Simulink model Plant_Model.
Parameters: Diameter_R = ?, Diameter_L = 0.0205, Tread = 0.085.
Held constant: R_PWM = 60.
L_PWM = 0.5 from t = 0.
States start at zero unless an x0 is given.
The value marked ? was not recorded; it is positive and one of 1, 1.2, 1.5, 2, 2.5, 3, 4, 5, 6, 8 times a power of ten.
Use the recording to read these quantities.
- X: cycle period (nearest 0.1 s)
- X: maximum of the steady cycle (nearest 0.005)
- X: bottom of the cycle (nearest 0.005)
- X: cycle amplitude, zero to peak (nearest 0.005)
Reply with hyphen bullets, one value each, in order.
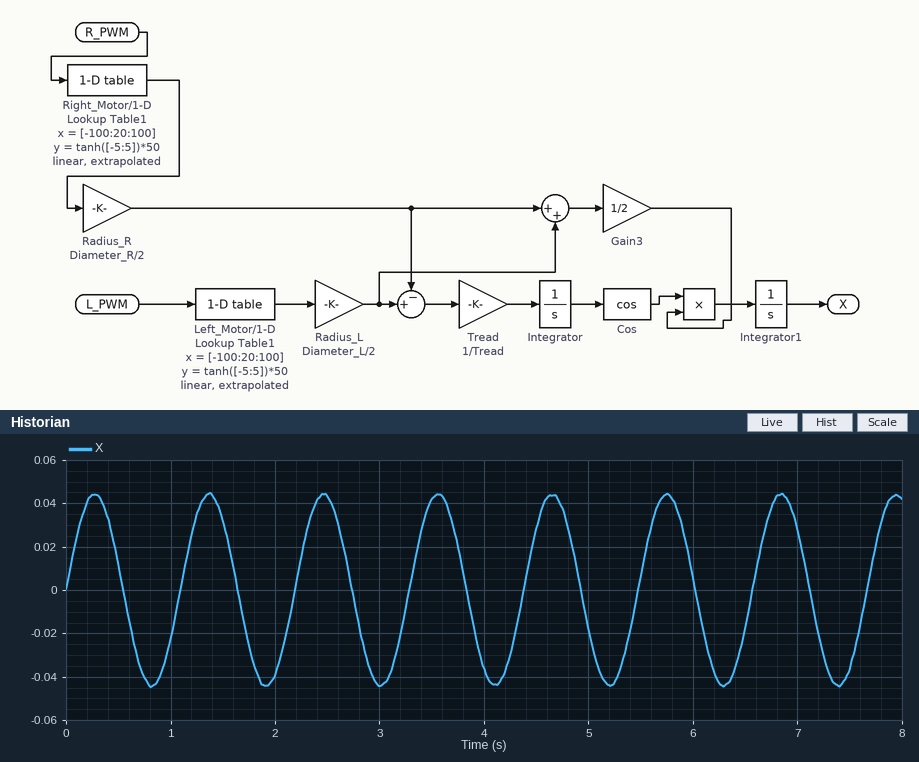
- 1.1 s
- 0.045
- -0.045
- 0.045
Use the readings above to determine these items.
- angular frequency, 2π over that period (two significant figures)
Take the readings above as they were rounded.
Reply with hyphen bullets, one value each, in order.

- 5.7 rad/s
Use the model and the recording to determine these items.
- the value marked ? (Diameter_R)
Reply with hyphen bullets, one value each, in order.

- 0.02
